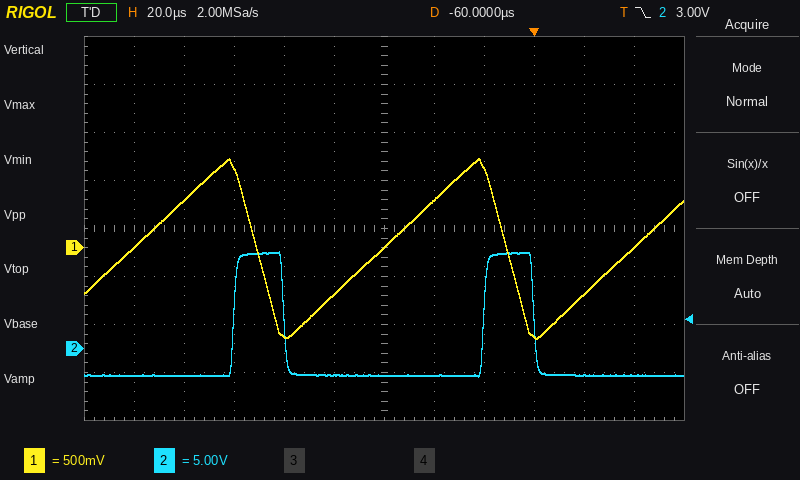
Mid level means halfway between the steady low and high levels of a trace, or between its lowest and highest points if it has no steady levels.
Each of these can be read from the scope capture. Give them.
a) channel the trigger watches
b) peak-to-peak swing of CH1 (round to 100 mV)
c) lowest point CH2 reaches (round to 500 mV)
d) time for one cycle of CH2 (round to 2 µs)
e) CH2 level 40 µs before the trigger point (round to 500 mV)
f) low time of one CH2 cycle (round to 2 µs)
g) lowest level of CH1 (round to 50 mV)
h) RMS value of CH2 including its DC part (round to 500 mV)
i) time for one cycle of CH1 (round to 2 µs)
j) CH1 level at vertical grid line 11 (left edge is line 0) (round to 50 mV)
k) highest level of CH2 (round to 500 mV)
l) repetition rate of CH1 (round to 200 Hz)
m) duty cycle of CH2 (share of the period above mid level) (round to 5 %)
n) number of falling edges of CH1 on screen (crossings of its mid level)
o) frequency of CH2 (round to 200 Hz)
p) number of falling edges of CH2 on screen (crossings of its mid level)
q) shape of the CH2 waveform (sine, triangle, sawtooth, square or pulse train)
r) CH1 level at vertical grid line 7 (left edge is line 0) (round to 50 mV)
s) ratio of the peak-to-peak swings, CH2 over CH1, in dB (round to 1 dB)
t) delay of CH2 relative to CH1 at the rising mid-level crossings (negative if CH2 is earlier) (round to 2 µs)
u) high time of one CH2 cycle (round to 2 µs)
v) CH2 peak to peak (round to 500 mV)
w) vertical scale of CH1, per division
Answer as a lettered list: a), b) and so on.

a) CH2
b) 1.90 V
c) -3.0 V
d) 100 µs
e) -3.0 V
f) 80 µs
g) -950 mV
h) 5.0 V
i) 100 µs
j) 0 mV
k) 10.0 V
l) 10.0 kHz
m) 20 %
n) 2
o) 10.0 kHz
p) 2
q) pulse train
r) 500 mV
s) 17 dB
t) +40 µs
u) 20 µs
v) 13.0 V
w) 500 mV
